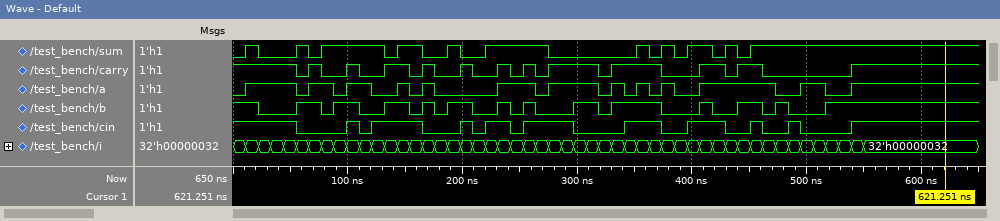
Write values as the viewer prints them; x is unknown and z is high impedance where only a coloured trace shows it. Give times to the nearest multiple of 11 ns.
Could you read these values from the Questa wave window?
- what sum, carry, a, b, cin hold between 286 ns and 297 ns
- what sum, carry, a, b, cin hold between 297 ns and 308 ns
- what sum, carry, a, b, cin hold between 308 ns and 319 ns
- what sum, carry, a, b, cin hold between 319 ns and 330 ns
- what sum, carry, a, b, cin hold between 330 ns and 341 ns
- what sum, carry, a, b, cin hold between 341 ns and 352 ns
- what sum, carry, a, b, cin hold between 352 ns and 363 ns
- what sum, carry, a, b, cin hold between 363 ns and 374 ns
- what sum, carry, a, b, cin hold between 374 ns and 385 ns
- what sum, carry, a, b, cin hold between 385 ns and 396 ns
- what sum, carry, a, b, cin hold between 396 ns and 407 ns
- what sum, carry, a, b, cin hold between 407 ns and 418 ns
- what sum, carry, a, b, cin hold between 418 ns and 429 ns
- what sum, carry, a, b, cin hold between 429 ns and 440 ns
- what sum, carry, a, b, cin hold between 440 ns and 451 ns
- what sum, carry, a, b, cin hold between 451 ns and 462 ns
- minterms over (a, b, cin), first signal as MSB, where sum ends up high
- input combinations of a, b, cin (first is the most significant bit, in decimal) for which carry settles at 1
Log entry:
sum=0, carry=1, a=1, b=0, cin=1
sum=0, carry=1, a=1, b=1, cin=0
sum=0, carry=1, a=1, b=1, cin=0
sum=0, carry=0, a=0, b=0, cin=0
sum=0, carry=1, a=1, b=1, cin=0
sum=0, carry=1, a=0, b=1, cin=1
sum=1, carry=1, a=1, b=1, cin=1
sum=0, carry=1, a=0, b=1, cin=1
sum=1, carry=0, a=1, b=0, cin=0
sum=0, carry=0, a=0, b=0, cin=0
sum=1, carry=0, a=0, b=0, cin=1
sum=1, carry=1, a=1, b=1, cin=1
sum=0, carry=1, a=1, b=0, cin=1
sum=1, carry=0, a=1, b=0, cin=0
sum=0, carry=1, a=1, b=1, cin=0
sum=1, carry=1, a=1, b=1, cin=1
1, 2, 4, 7
3, 5, 6, 7
